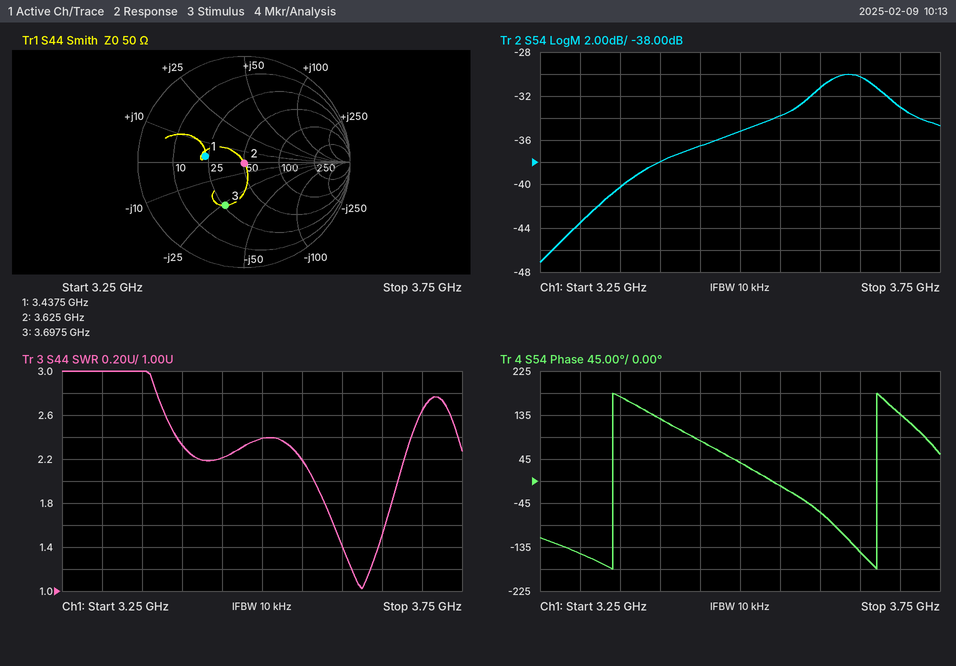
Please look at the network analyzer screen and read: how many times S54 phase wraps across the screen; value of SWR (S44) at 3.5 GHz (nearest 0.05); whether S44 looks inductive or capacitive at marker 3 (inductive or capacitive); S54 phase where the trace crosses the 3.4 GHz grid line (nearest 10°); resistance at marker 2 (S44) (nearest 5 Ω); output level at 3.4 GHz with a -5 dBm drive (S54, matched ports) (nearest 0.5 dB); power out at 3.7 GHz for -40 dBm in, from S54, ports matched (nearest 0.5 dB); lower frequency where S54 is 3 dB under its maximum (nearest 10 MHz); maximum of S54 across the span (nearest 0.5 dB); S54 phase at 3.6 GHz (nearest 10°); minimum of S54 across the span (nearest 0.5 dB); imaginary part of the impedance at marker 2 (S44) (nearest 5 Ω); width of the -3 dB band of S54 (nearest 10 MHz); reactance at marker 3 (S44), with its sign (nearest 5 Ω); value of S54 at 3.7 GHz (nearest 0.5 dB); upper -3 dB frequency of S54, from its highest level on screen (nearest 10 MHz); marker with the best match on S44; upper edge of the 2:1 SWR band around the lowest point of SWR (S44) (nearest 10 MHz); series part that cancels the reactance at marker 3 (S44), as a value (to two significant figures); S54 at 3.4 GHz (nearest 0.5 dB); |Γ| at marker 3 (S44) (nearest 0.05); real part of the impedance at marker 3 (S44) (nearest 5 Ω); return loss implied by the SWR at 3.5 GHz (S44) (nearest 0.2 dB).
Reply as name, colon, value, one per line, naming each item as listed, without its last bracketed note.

how many times S54 phase wraps across the screen: 2
value of SWR (S44) at 3.5 GHz: 2.40
whether S44 looks inductive or capacitive at marker 3: capacitive
S54 phase where the trace crosses the 3.4 GHz grid line: 130°
resistance at marker 2 (S44): 50 Ω
output level at 3.4 GHz with a -5 dBm drive (S54, matched ports): -43.0 dBm
power out at 3.7 GHz for -40 dBm in, from S54, ports matched: -73.0 dBm
lower frequency where S54 is 3 dB under its maximum: 3.57 GHz
maximum of S54 across the span: -30.0 dB
S54 phase at 3.6 GHz: -60°
minimum of S54 across the span: -47.0 dB
imaginary part of the impedance at marker 2 (S44): 0 Ω
width of the -3 dB band of S54: 130 MHz
reactance at marker 3 (S44), with its sign: -25 Ω
value of S54 at 3.7 GHz: -33.0 dB
upper -3 dB frequency of S54, from its highest level on screen: 3.70 GHz
marker with the best match on S44: marker 2
upper edge of the 2:1 SWR band around the lowest point of SWR (S44): 3.67 GHz
series part that cancels the reactance at marker 3 (S44), as a value: 1.1 nH
S54 at 3.4 GHz: -38.0 dB
|Γ| at marker 3 (S44): 0.45
real part of the impedance at marker 3 (S44): 25 Ω
return loss implied by the SWR at 3.5 GHz (S44): 7.8 dB
